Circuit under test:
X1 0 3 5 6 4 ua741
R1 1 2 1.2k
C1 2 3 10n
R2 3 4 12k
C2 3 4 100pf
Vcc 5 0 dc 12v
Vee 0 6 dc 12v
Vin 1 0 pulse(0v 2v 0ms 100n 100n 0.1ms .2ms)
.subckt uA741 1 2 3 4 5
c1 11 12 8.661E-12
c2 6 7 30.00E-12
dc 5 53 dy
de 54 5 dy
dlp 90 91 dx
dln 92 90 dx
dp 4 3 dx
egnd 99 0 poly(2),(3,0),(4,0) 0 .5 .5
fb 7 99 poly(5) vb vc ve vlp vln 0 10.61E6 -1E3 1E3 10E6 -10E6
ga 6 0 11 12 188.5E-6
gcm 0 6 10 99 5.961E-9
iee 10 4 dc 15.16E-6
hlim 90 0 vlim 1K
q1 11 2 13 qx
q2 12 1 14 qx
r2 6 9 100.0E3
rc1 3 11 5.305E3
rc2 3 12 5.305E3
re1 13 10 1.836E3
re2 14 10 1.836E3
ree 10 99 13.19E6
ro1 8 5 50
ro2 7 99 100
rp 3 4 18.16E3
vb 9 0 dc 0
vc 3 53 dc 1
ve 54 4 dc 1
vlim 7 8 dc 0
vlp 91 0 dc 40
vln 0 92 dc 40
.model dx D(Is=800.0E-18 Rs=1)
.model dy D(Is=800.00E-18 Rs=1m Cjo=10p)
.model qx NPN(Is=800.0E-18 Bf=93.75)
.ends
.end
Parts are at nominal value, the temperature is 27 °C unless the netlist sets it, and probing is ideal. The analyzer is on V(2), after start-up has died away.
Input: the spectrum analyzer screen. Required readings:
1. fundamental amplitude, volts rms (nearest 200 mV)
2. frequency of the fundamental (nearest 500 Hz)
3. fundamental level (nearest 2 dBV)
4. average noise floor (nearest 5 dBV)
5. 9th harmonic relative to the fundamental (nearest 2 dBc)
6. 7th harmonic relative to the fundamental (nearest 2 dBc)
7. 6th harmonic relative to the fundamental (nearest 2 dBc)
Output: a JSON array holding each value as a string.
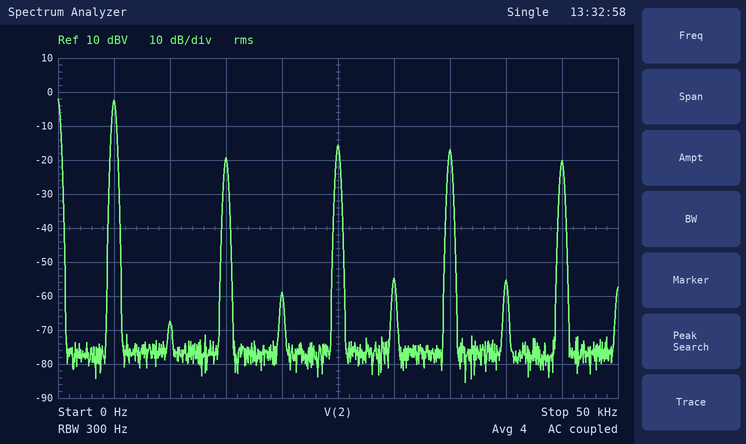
["800 mV", "5.0 kHz", "-2 dBV", "-75 dBV", "-18 dBc", "-14 dBc", "-52 dBc"]
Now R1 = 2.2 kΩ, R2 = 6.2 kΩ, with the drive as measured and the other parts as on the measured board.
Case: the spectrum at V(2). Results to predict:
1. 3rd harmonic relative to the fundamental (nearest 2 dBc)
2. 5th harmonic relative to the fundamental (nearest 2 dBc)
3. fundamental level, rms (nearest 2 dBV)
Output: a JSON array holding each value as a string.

["-22 dBc", "-24 dBc", "-4 dBV"]
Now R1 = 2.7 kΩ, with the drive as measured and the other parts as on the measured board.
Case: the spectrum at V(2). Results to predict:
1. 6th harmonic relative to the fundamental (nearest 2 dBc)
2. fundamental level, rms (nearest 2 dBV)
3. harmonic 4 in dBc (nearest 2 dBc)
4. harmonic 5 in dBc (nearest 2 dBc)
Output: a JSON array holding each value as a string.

["-54 dBc", "-4 dBV", "-60 dBc", "-16 dBc"]
